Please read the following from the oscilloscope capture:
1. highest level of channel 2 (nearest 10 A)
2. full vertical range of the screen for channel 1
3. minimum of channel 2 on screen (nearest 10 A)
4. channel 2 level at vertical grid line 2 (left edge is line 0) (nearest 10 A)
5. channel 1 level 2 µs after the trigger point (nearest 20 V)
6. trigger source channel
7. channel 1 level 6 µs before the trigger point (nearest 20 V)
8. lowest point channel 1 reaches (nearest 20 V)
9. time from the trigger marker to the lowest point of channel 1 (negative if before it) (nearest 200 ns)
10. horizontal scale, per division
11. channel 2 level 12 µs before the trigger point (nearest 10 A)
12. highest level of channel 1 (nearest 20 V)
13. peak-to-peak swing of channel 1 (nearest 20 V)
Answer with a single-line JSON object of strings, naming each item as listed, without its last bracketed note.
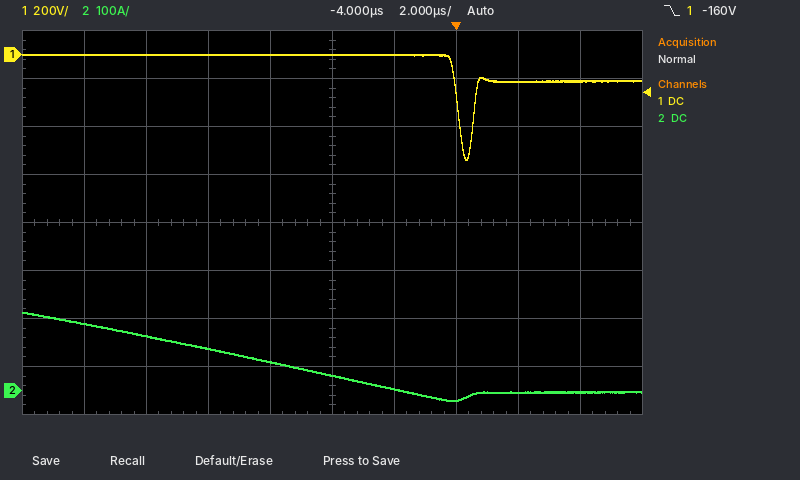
{"highest level of channel 2": "160 A", "full vertical range of the screen for channel 1": "1.6 kV", "minimum of channel 2 on screen": "-20 A", "channel 2 level at vertical grid line 2 (left edge is line 0)": "110 A", "channel 1 level 2 µs after the trigger point": "-120 V", "trigger source channel": "channel 1", "channel 1 level 6 µs before the trigger point": "0 V", "lowest point channel 1 reaches": "-440 V", "time from the trigger marker to the lowest point of channel 1 (negative if before it)": "+400 ns", "horizontal scale, per division": "2 µs", "channel 2 level 12 µs before the trigger point": "140 A", "highest level of channel 1": "0 V", "peak-to-peak swing of channel 1": "440 V"}
